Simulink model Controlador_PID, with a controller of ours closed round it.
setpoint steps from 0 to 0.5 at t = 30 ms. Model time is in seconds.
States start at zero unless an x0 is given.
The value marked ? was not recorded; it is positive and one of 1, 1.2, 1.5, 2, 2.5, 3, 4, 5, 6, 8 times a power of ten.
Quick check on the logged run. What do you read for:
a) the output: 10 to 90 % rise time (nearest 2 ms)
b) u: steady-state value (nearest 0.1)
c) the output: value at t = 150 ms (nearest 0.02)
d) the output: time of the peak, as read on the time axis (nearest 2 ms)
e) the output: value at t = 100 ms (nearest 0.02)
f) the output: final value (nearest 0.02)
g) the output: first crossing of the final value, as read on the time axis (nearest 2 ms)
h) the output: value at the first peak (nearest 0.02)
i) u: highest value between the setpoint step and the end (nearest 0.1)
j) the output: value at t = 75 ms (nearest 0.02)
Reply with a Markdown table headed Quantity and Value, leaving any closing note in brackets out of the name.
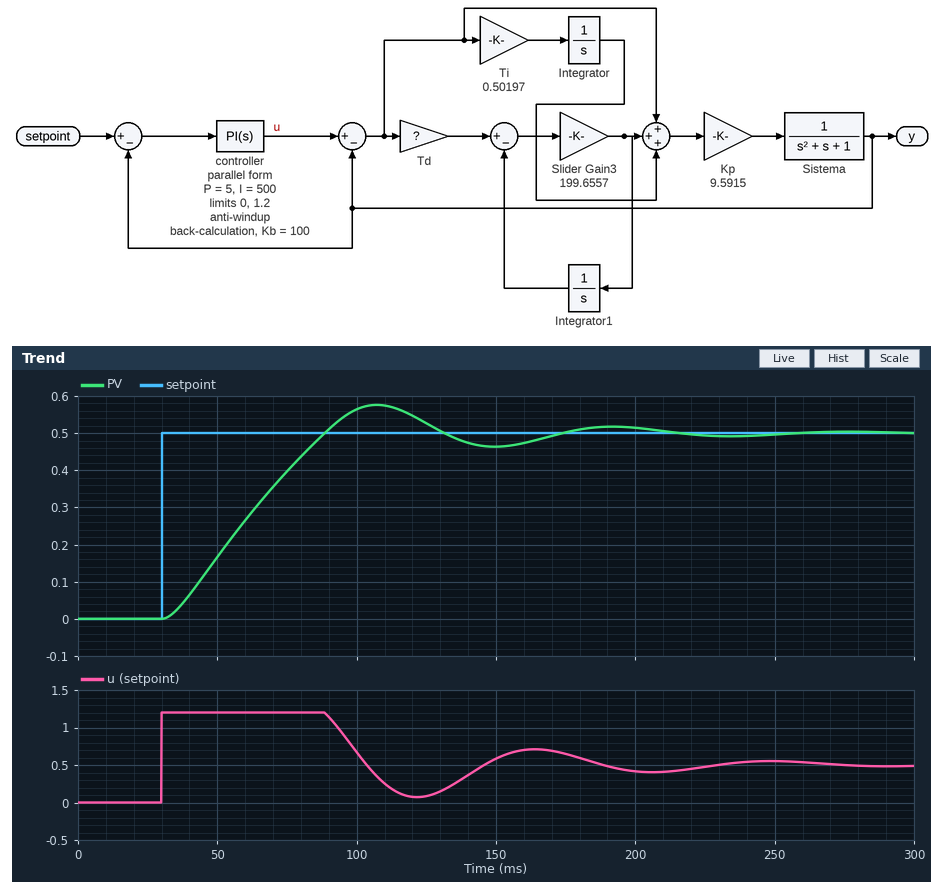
| Quantity | Value |
|---|---|
| the output: 10 to 90 % rise time | 44 ms |
| u: steady-state value | 0.5 |
| the output: value at t = 150 ms | 0.46 |
| the output: time of the peak, as read on the time axis | 108 ms |
| the output: value at t = 100 ms | 0.56 |
| the output: final value | 0.50 |
| the output: first crossing of the final value, as read on the time axis | 88 ms |
| the output: value at the first peak | 0.58 |
| u: highest value between the setpoint step and the end | 1.2 |
| the output: value at t = 75 ms | 0.40 |
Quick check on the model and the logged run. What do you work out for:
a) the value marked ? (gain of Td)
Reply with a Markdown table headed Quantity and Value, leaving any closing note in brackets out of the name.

| Quantity | Value |
|---|---|
| the value marked ? | 1 |
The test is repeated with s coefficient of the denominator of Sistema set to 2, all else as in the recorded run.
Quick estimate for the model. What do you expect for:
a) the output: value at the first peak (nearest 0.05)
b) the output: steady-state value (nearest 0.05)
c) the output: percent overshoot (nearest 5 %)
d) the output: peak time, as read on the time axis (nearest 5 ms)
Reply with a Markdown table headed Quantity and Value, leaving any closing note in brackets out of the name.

| Quantity | Value |
|---|---|
| the output: value at the first peak | 0.55 |
| the output: steady-state value | 0.50 |
| the output: percent overshoot | 15 % |
| the output: peak time, as read on the time axis | 110 ms |
